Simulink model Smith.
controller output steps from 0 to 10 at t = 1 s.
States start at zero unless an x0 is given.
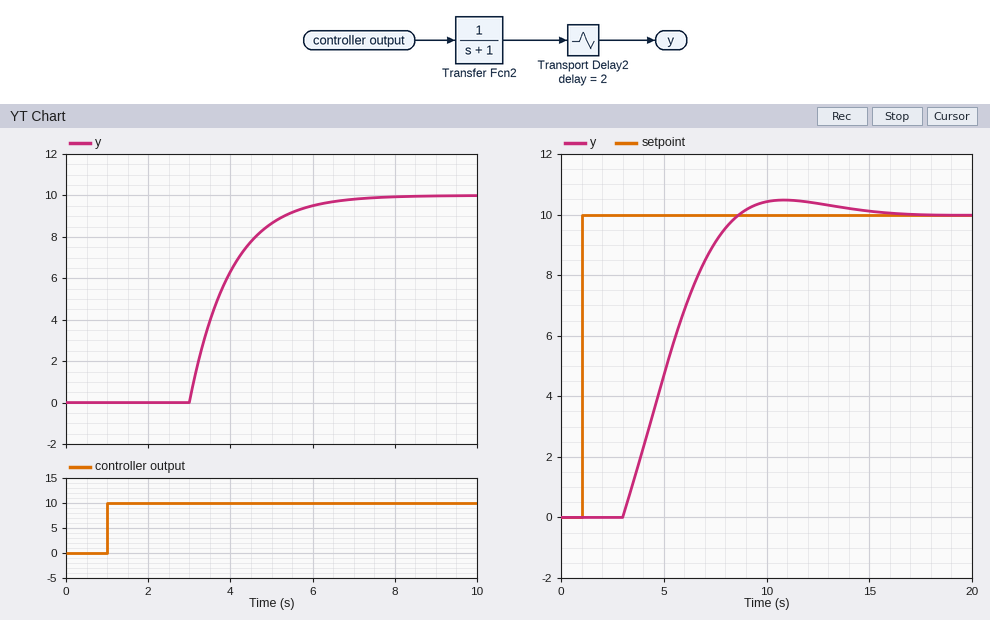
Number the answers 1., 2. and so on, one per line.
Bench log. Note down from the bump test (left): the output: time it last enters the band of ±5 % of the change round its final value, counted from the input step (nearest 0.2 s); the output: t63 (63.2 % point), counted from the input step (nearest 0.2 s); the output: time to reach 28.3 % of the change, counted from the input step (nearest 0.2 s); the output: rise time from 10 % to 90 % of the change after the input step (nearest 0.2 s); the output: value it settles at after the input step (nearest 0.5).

1. 5.0 s
2. 3.0 s
3. 2.4 s
4. 2.2 s
5. 10.0
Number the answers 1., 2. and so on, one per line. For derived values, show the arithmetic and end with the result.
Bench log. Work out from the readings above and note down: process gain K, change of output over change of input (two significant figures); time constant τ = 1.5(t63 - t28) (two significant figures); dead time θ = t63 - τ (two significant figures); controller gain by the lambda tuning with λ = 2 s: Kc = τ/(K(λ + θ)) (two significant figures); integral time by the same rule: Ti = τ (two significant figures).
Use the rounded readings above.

1. (10 - 0) / 10 = 1.0
2. 1.5 × (3 - 2.4) = 0.90 s
3. 3 - 0.9 = 2.1 s
4. 0.9 / (1 × (2 + 2.1)) = 0.22
5. 0.90 s
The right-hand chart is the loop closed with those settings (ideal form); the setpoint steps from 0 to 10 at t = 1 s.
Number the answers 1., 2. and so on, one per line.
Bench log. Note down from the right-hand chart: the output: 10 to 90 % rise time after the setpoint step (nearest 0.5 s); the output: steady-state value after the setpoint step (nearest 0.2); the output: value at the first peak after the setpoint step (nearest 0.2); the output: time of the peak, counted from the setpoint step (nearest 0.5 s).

1. 4.0 s
2. 10.0
3. 10.4
4. 10.0 s
